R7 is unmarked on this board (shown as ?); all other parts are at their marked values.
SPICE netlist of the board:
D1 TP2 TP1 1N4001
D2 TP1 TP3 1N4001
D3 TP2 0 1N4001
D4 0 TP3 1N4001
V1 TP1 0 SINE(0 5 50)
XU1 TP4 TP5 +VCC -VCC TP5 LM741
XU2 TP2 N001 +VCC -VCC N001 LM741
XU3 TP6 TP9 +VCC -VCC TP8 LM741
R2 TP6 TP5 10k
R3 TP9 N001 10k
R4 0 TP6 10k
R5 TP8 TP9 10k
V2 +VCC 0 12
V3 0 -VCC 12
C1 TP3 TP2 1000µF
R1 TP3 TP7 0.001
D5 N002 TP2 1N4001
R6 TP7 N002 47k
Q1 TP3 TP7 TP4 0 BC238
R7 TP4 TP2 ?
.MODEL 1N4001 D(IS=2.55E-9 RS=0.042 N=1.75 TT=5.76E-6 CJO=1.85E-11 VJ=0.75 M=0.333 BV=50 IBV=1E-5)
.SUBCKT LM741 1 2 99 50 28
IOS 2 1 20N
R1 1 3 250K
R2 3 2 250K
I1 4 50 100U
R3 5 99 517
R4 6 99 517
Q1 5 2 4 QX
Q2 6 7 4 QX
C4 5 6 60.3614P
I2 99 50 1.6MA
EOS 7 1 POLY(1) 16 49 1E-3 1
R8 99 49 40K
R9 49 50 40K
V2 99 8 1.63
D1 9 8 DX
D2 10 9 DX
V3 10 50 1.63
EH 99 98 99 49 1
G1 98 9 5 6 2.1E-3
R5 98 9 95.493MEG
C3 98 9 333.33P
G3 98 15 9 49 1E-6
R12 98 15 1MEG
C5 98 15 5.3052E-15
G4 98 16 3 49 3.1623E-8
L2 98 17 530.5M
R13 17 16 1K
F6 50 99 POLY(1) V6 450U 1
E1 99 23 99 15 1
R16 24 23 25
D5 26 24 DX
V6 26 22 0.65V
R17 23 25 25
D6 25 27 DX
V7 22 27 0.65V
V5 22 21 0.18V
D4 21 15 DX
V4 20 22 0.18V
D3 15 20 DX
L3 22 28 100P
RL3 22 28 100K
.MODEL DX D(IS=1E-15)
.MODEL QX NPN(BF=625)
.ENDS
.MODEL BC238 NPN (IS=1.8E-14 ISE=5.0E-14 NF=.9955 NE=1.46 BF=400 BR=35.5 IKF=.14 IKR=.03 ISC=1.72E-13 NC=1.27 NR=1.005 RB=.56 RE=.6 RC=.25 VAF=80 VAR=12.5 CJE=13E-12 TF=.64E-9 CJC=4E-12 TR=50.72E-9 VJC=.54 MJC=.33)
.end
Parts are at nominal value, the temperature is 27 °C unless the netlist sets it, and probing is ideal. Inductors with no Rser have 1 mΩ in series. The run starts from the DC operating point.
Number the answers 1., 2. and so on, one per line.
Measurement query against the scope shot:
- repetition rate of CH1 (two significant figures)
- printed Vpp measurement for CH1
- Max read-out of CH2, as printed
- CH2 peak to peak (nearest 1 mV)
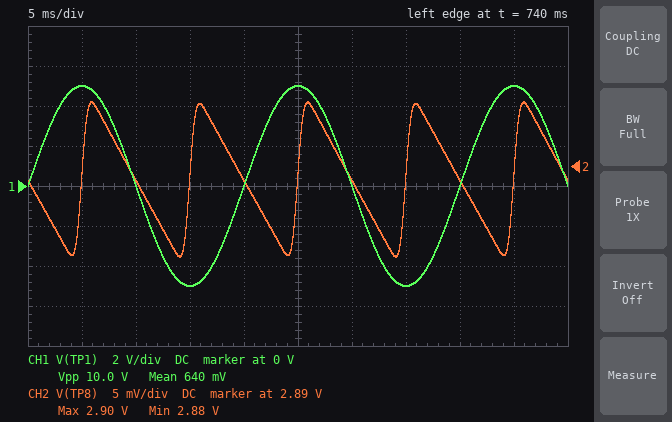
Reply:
1. 50 Hz
2. 10.0 V
3. 2.90 V
4. 19 mV
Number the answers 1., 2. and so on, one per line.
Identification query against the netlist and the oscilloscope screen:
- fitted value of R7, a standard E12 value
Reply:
1. 1.2 kΩ
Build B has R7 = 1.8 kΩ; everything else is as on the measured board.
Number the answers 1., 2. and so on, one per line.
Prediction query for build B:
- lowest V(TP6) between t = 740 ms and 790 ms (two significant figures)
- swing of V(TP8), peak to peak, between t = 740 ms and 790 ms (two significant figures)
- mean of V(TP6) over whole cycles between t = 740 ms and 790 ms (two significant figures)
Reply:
1. -680 mV
2. 13 mV
3. 310 mV
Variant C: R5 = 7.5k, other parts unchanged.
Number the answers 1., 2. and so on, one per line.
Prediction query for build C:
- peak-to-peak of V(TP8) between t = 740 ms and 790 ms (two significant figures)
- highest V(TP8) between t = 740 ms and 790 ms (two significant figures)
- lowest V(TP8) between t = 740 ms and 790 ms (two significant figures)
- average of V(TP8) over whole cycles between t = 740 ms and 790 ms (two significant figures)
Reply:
1. 630 mV
2. 2.6 V
3. 2.0 V
4. 2.2 V
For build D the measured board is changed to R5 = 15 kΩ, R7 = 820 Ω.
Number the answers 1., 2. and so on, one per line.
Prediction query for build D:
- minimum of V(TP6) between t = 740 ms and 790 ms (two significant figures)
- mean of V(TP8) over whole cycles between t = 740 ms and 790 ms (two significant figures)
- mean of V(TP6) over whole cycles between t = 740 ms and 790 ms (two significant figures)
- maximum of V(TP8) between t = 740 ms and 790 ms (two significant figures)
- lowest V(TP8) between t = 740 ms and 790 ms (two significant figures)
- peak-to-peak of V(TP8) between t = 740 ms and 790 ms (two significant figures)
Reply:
1. -710 mV
2. 4.1 V
3. 290 mV
4. 4.6 V
5. 3.4 V
6. 1.3 V
